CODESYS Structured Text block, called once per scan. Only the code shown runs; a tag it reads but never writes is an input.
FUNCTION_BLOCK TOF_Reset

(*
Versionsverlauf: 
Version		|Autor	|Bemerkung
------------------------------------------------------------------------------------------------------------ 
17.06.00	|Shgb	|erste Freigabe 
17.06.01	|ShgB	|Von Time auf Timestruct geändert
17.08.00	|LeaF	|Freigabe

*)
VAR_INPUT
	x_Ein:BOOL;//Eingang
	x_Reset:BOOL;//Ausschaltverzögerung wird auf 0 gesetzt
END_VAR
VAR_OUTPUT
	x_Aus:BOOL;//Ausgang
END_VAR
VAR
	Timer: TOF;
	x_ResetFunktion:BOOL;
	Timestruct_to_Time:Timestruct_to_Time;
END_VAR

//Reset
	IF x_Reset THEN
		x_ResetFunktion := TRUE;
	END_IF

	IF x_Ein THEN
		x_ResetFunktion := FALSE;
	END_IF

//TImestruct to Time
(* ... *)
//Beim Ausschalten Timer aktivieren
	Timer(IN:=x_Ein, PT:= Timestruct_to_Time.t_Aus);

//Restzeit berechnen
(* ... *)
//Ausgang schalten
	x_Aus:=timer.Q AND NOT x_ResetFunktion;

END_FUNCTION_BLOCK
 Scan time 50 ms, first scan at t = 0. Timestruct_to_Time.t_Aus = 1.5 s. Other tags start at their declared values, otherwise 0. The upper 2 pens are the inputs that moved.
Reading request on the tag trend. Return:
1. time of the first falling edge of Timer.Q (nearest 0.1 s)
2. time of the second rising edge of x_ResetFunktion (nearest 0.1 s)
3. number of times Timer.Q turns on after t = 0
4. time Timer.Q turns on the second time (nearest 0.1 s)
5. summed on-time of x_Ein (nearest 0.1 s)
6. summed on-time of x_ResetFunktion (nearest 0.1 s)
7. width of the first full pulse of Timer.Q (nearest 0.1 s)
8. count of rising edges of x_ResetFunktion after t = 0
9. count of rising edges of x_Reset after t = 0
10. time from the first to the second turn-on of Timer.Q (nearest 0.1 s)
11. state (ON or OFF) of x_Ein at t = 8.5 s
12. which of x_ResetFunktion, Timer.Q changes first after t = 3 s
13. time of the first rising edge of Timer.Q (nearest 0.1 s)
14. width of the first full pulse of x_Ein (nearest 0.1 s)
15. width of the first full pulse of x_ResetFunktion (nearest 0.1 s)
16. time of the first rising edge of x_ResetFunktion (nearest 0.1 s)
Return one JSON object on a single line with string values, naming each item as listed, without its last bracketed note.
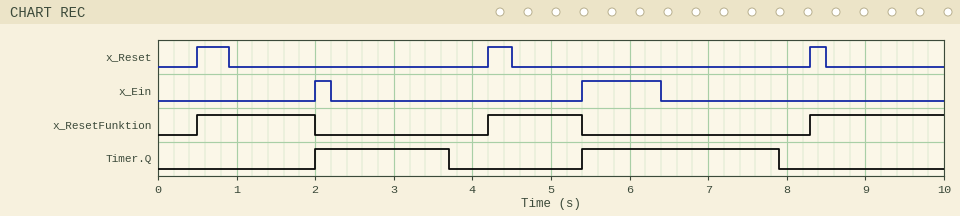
{"time of the first falling edge of Timer.Q": "3.7 s", "time of the second rising edge of x_ResetFunktion": "4.2 s", "number of times Timer.Q turns on after t = 0": "2", "time Timer.Q turns on the second time": "5.4 s", "summed on-time of x_Ein": "1.2 s", "summed on-time of x_ResetFunktion": "4.4 s", "width of the first full pulse of Timer.Q": "1.7 s", "count of rising edges of x_ResetFunktion after t = 0": "3", "count of rising edges of x_Reset after t = 0": "3", "time from the first to the second turn-on of Timer.Q": "3.4 s", "state (ON or OFF) of x_Ein at t = 8.5 s": "OFF", "which of x_ResetFunktion, Timer.Q changes first after t = 3 s": "Timer.Q", "time of the first rising edge of Timer.Q": "2.0 s", "width of the first full pulse of x_Ein": "0.2 s", "width of the first full pulse of x_ResetFunktion": "1.5 s", "time of the first rising edge of x_ResetFunktion": "0.5 s"}
